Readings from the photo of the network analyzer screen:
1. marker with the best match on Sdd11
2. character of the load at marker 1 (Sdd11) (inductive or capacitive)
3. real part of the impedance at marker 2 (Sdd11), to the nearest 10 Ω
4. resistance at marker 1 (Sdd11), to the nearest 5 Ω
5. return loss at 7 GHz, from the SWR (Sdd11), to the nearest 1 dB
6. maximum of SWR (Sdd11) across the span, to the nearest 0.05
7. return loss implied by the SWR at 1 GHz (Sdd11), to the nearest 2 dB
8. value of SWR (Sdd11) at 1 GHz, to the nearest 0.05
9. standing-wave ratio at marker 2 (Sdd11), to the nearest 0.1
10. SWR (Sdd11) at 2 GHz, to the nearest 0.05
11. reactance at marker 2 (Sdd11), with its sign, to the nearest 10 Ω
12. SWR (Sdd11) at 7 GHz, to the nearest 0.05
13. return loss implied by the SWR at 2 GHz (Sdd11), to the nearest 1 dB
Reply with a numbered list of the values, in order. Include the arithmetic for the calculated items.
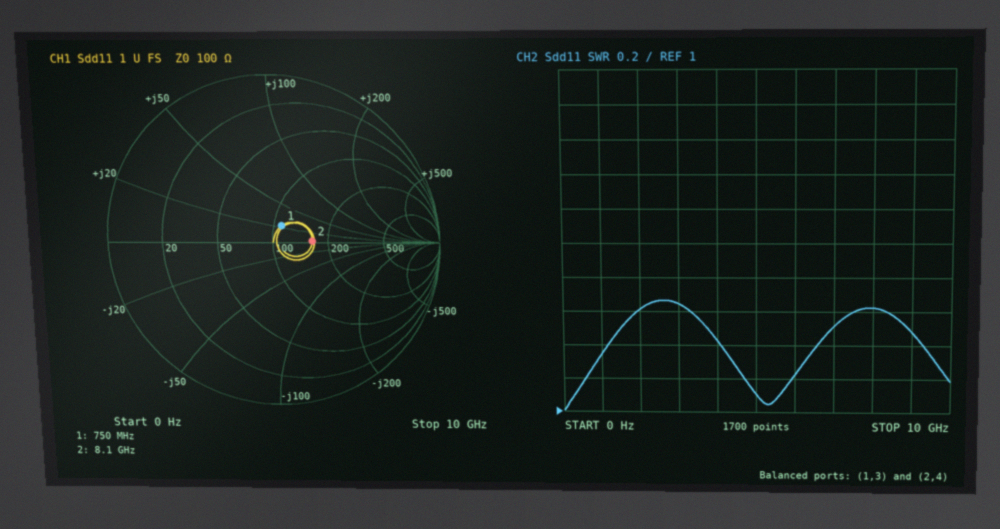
1. marker 1
2. inductive
3. 160 Ω
4. 110 Ω
5. −20 log10((1.5 − 1)/(1.5 + 1)) ≈ 14 dB
6. 1.65
7. −20 log10((1.35 − 1)/(1.35 + 1)) ≈ 16 dB
8. 1.35
9. 1.6
10. 1.60
11. 0 Ω
12. 1.50
13. −20 log10((1.6 − 1)/(1.6 + 1)) ≈ 13 dB
